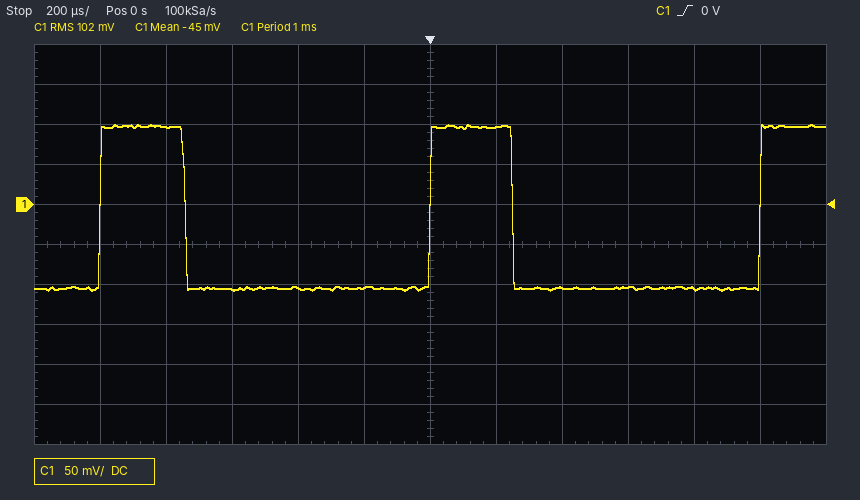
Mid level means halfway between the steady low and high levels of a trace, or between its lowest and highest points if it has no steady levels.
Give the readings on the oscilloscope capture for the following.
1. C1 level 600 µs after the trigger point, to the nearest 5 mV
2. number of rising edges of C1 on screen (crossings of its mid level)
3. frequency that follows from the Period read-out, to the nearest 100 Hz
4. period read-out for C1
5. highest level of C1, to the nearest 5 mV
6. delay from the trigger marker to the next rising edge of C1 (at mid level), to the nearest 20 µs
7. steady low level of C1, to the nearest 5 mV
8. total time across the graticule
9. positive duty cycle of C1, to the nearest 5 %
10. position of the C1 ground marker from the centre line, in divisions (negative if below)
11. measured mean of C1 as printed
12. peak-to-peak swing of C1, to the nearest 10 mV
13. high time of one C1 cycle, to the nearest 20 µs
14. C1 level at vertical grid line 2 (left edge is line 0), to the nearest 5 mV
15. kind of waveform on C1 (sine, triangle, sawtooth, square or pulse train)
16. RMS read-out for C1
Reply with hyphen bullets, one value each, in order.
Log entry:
- -105 mV
- 3
- 1.0 kHz
- 1 ms
- 100 mV
- 1.00 ms
- -105 mV
- 2.4 ms
- 25 %
- +1.0 div
- -45 mV
- 210 mV
- 260 µs
- 95 mV
- pulse train
- 102 mV
